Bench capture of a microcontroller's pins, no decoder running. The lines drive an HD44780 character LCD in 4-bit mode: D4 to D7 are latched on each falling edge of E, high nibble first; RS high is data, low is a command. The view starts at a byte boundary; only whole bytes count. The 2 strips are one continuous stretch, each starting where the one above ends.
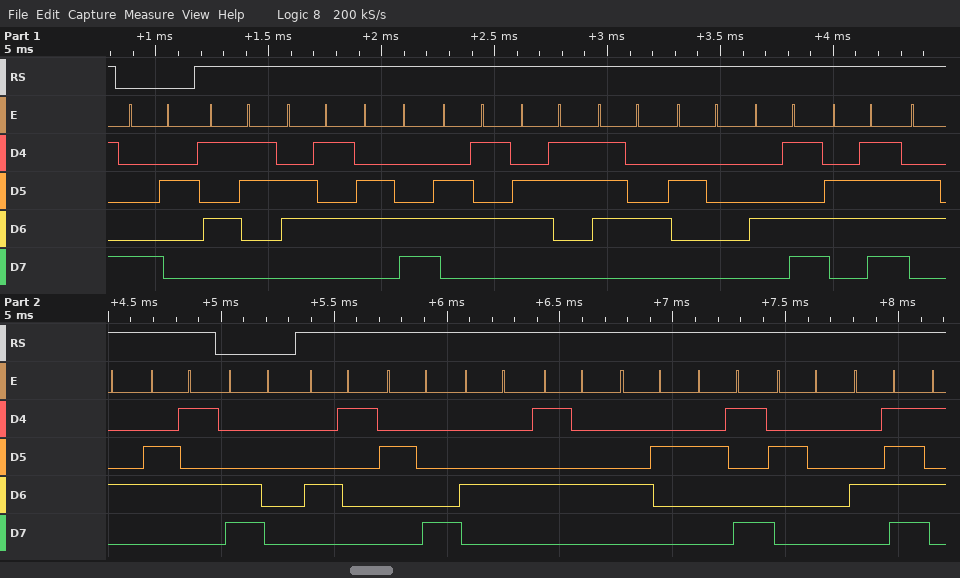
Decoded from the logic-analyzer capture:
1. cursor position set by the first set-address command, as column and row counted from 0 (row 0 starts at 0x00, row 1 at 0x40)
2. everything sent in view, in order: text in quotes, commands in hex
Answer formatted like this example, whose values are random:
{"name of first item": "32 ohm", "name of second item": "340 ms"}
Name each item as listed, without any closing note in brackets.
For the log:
{"cursor position set by the first set-address command, as column and row counted from 0": "column 2, row 0", "everything sent in view, in order: text in quotes, commands in hex": "0x82 \"Select Mode\" 0xC0 \"A(DTB) O\""}
